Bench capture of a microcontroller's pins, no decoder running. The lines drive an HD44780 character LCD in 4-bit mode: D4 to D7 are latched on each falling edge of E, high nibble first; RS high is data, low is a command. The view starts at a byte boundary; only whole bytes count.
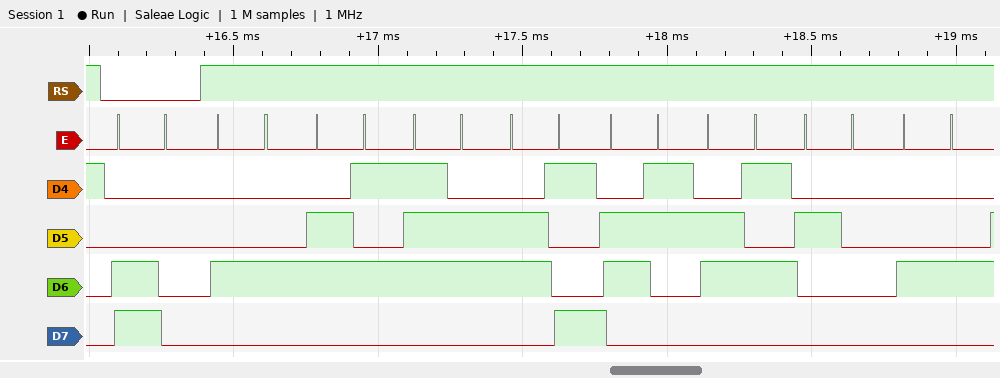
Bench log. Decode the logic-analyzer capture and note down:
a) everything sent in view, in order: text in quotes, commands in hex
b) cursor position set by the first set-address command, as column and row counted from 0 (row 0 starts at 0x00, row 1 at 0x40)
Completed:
0xC0 "Device D"
column 0, row 1
